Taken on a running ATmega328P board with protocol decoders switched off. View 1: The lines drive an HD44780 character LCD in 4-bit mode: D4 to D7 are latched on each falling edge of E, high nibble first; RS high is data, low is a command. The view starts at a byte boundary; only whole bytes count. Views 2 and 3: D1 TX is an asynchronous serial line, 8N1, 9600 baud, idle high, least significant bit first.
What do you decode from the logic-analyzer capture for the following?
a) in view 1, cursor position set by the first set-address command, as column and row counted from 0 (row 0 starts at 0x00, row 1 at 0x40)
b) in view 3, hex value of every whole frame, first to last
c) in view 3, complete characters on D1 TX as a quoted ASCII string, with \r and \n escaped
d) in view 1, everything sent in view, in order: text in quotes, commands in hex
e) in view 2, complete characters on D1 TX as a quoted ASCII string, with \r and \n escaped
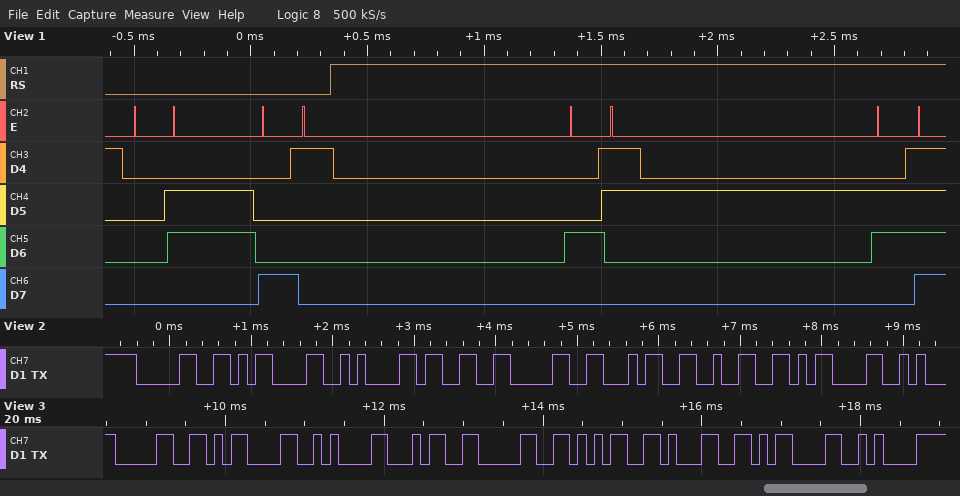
column 1, row 0
30 0D 0A 34 30 35 31 0D 0A
"0\r\n4051\r\n"
0x06 0x81 "Co"
"0\r\n3042\r"
